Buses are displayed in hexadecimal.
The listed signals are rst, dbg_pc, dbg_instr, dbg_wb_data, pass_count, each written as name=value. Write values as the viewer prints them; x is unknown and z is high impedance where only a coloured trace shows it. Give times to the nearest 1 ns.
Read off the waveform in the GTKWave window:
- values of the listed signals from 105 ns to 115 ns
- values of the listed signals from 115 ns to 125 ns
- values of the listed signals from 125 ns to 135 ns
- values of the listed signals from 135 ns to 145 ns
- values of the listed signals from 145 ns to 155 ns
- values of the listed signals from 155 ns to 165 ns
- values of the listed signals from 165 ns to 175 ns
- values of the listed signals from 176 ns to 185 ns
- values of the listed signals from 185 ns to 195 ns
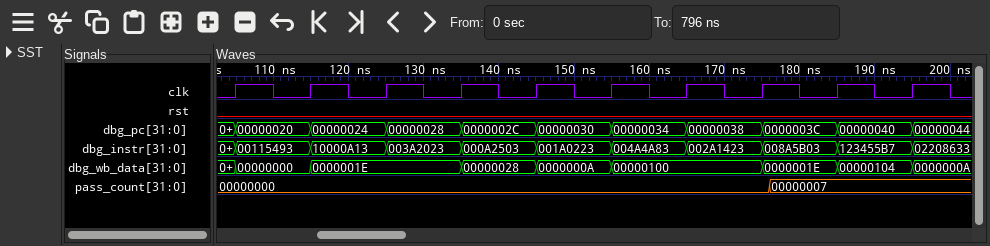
rst=0, dbg_pc=00000020, dbg_instr=00115493, dbg_wb_data=00000000, pass_count=00000000
rst=0, dbg_pc=00000024, dbg_instr=10000A13, dbg_wb_data=0000001E, pass_count=00000000
rst=0, dbg_pc=00000028, dbg_instr=003A2023, dbg_wb_data=0000001E, pass_count=00000000
rst=0, dbg_pc=0000002C, dbg_instr=000A2503, dbg_wb_data=00000028, pass_count=00000000
rst=0, dbg_pc=00000030, dbg_instr=001A0223, dbg_wb_data=0000000A, pass_count=00000000
rst=0, dbg_pc=00000034, dbg_instr=004A4A83, dbg_wb_data=00000100, pass_count=00000000
rst=0, dbg_pc=00000038, dbg_instr=002A1423, dbg_wb_data=00000100, pass_count=00000000
rst=0, dbg_pc=0000003C, dbg_instr=008A5B03, dbg_wb_data=0000001E, pass_count=00000007
rst=0, dbg_pc=00000040, dbg_instr=123455B7, dbg_wb_data=00000104, pass_count=00000007
